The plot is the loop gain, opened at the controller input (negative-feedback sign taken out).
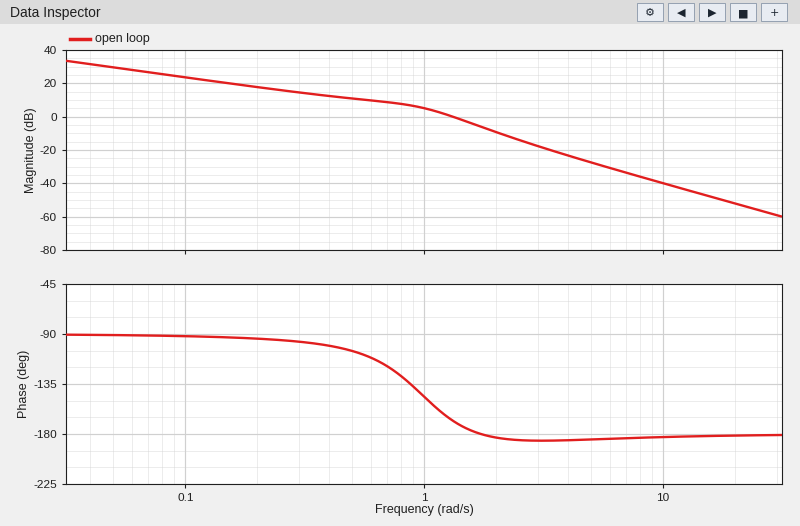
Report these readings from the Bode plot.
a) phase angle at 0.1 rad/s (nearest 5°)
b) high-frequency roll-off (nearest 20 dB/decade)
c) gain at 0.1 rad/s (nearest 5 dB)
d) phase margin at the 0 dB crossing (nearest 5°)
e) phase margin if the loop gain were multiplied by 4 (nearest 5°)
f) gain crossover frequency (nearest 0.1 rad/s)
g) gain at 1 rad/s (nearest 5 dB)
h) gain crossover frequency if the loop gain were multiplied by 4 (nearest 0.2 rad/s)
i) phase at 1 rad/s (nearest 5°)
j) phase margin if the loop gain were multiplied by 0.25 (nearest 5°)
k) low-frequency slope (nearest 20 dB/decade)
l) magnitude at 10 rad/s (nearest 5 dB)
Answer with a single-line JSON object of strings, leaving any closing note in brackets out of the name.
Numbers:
{"phase angle at 0.1 rad/s": "-90°", "high-frequency roll-off": "-40 dB/decade", "gain at 0.1 rad/s": "25 dB", "phase margin at the 0 dB crossing": "10°", "phase margin if the loop gain were multiplied by 4": "-5°", "gain crossover frequency": "1.3 rad/s", "gain at 1 rad/s": "5 dB", "gain crossover frequency if the loop gain were multiplied by 4": "2.2 rad/s", "phase at 1 rad/s": "-145°", "phase margin if the loop gain were multiplied by 0.25": "80°", "low-frequency slope": "-20 dB/decade", "magnitude at 10 rad/s": "-40 dB"}
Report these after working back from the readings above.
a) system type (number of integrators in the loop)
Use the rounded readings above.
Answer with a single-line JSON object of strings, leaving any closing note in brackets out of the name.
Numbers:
{"system type": "1"}
